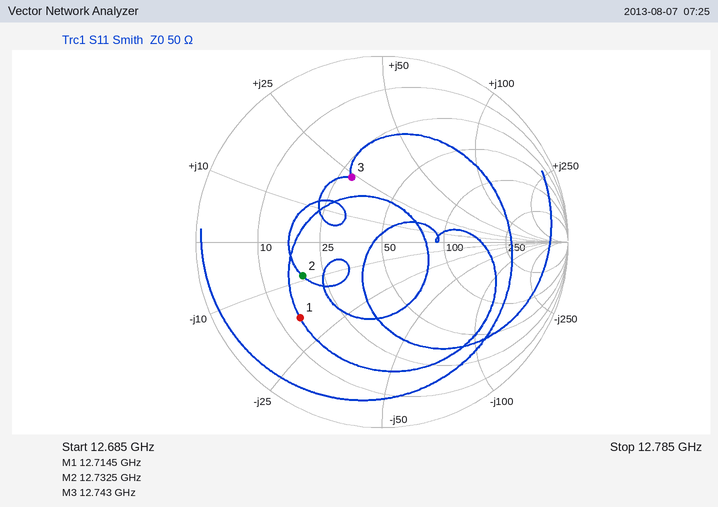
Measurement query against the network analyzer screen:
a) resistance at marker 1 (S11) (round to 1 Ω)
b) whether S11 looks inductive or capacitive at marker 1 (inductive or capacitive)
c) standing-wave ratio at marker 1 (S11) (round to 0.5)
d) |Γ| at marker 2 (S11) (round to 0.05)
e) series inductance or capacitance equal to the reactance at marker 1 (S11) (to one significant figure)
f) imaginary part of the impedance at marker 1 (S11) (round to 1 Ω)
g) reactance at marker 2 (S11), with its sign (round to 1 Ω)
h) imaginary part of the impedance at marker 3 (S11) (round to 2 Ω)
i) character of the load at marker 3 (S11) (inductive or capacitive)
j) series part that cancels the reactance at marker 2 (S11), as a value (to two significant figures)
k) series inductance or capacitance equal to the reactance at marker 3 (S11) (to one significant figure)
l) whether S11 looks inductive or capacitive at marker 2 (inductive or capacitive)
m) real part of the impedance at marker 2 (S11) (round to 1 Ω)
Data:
14 Ω
capacitive
4.0
0.45
700 fF
-18 Ω
-9 Ω
+24 Ω
inductive
110 pH
300 pH
capacitive
19 Ω
